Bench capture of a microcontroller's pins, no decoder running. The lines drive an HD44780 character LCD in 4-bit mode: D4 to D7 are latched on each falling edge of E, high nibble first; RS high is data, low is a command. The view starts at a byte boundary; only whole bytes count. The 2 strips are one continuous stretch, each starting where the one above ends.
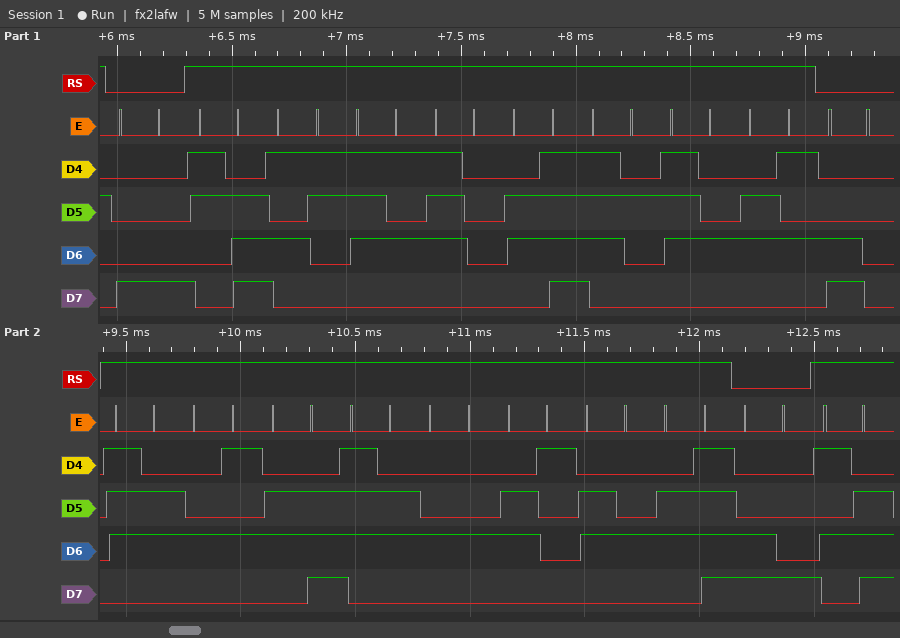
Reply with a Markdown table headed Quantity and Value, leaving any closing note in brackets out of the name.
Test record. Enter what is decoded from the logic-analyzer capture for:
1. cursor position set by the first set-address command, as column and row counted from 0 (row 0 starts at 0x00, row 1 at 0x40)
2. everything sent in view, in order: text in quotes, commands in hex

| Quantity | Value |
|---|---|
| cursor position set by the first set-address command, as column and row counted from 0 | column 8, row 0 |
| everything sent in view, in order: text in quotes, commands in hex | 0x88 ">Suporte" 0xC0 "vEnvDado" 0xC8 "^" |
